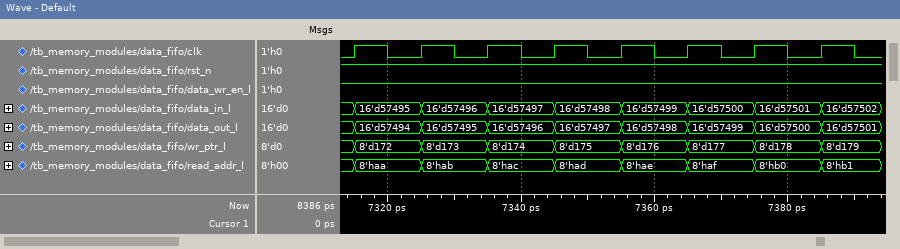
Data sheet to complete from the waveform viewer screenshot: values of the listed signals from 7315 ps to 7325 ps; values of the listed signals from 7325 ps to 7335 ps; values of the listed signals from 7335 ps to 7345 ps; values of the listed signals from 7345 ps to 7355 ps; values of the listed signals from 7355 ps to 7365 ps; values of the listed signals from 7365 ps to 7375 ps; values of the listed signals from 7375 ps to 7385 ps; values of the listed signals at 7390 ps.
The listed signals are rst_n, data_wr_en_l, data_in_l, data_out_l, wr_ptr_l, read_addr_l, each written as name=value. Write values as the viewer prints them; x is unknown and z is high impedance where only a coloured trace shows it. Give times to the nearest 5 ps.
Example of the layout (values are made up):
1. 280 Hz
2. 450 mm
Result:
1. rst_n=1, data_wr_en_l=1, data_in_l=16'd57495, data_out_l=16'd57494, wr_ptr_l=8'd172, read_addr_l=8'haa
2. rst_n=1, data_wr_en_l=1, data_in_l=16'd57496, data_out_l=16'd57495, wr_ptr_l=8'd173, read_addr_l=8'hab
3. rst_n=1, data_wr_en_l=1, data_in_l=16'd57497, data_out_l=16'd57496, wr_ptr_l=8'd174, read_addr_l=8'hac
4. rst_n=1, data_wr_en_l=1, data_in_l=16'd57498, data_out_l=16'd57497, wr_ptr_l=8'd175, read_addr_l=8'had
5. rst_n=1, data_wr_en_l=1, data_in_l=16'd57499, data_out_l=16'd57498, wr_ptr_l=8'd176, read_addr_l=8'hae
6. rst_n=1, data_wr_en_l=1, data_in_l=16'd57500, data_out_l=16'd57499, wr_ptr_l=8'd177, read_addr_l=8'haf
7. rst_n=1, data_wr_en_l=1, data_in_l=16'd57501, data_out_l=16'd57500, wr_ptr_l=8'd178, read_addr_l=8'hb0
8. rst_n=1, data_wr_en_l=1, data_in_l=16'd57502, data_out_l=16'd57501, wr_ptr_l=8'd179, read_addr_l=8'hb1
